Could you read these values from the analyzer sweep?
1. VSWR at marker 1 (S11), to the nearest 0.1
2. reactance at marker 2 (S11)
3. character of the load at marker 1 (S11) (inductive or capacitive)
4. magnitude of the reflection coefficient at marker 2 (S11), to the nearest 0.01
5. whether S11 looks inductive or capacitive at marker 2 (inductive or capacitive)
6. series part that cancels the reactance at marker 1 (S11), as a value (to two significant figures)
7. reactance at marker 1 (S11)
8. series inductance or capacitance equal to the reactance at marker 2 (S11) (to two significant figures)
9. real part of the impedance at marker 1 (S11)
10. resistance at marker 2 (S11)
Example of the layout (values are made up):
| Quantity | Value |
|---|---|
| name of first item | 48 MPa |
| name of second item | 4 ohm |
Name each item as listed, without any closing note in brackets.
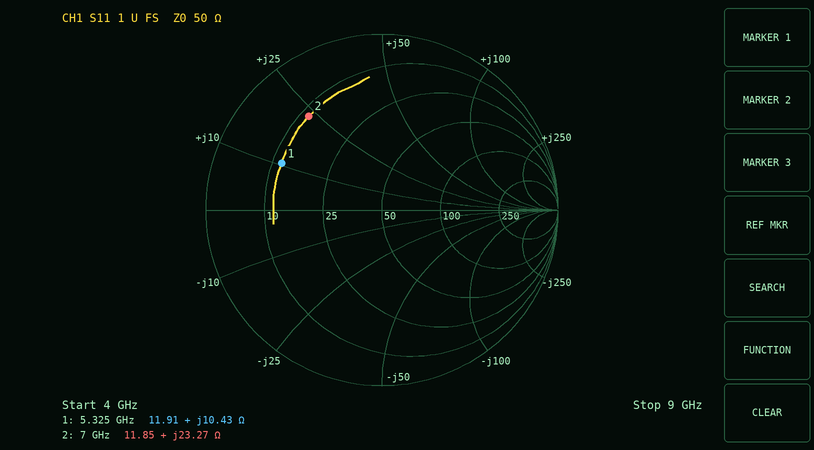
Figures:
| Quantity | Value |
|---|---|
| VSWR at marker 1 (S11), to the nearest 0.1 | 4.4 |
| reactance at marker 2 | +23.27 Ω |
| character of the load at marker 1 (S11) | inductive |
| magnitude of the reflection coefficient at marker 2 (S11), to the nearest 0.01 | 0.68 |
| whether S11 looks inductive or capacitive at marker 2 | inductive |
| series part that cancels the reactance at marker 1 (S11), as a value | 2.9 pF |
| reactance at marker 1 | +10.43 Ω |
| series inductance or capacitance equal to the reactance at marker 2 (S11) | 530 pH |
| real part of the impedance at marker 1 | 11.91 Ω |
| resistance at marker 2 | 11.85 Ω |
